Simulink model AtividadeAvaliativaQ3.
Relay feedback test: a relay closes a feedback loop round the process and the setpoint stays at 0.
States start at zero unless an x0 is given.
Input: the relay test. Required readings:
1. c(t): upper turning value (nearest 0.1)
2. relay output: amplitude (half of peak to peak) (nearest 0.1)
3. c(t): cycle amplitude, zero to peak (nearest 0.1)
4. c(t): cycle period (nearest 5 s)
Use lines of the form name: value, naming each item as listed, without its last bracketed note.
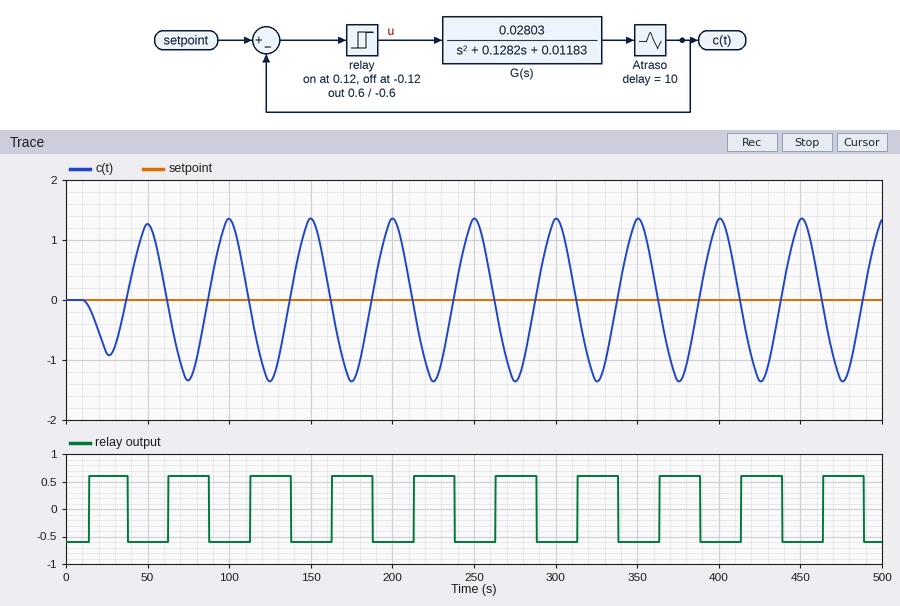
c(t): upper turning value: 1.4
relay output: amplitude (half of peak to peak): 0.6
c(t): cycle amplitude, zero to peak: 1.4
c(t): cycle period: 50 s
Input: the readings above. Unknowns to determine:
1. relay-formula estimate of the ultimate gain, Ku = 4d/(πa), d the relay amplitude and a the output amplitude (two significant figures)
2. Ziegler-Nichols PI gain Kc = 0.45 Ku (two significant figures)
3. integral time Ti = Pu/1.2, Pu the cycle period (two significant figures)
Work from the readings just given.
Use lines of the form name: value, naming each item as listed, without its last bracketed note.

relay-formula estimate of the ultimate gain, Ku = 4d/(πa), d the relay amplitude and a the output amplitude: 0.55
Ziegler-Nichols PI gain Kc = 0.45 Ku: 0.25
integral time Ti = Pu/1.2, Pu the cycle period: 42 s
